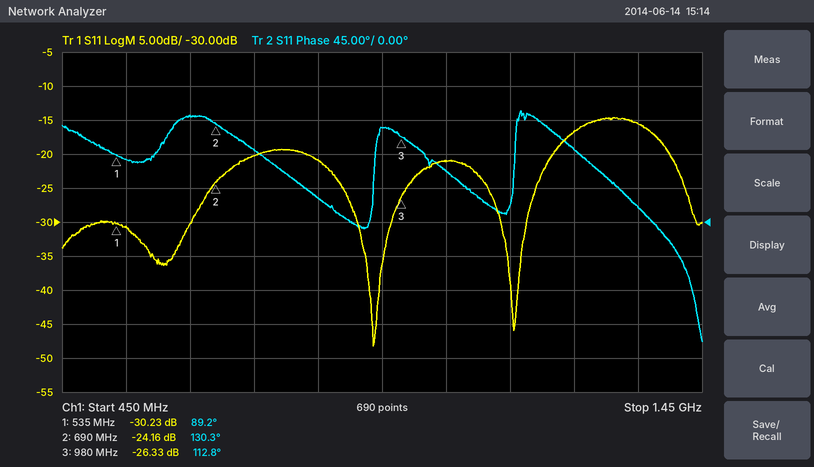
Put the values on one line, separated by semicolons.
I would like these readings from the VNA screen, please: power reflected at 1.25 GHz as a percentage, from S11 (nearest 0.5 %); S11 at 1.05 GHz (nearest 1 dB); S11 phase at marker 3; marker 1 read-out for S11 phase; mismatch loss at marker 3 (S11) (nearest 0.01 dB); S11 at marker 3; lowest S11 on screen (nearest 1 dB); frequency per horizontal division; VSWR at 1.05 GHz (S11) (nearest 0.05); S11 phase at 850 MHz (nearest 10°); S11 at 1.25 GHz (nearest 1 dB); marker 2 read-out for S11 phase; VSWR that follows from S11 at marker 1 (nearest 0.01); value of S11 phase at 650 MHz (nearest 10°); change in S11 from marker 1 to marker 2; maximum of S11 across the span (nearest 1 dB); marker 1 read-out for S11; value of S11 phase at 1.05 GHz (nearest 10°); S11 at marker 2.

2.0 %; -21 dB; 112.8°; 89.2°; 0.01 dB; -26.33 dB; -48 dB; 100 MHz; 1.20; 30°; -17 dB; 130.3°; 1.06; 140°; 6.07 dB; -15 dB; -30.23 dB; 70°; -24.16 dB
